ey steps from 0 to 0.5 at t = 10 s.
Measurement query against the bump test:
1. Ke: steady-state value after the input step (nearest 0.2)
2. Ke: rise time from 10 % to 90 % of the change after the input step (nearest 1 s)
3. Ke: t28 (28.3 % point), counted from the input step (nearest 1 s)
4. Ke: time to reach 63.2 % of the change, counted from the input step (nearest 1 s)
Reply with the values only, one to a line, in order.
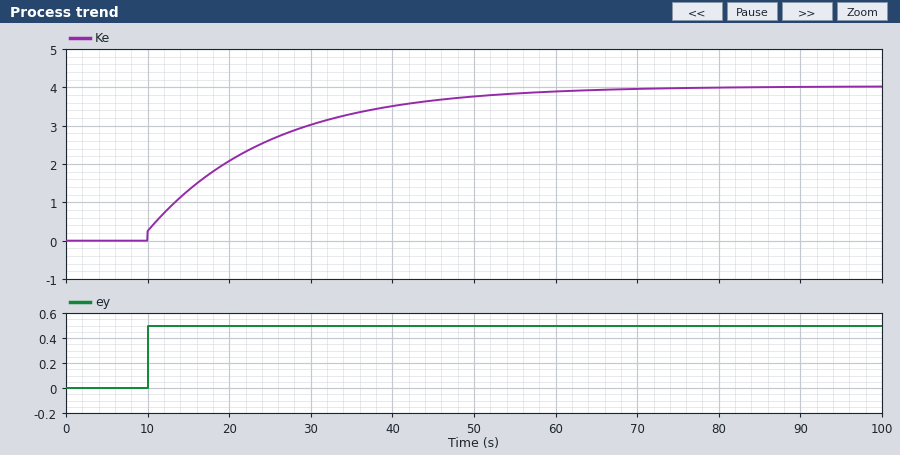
4.0
33 s
4 s
14 s
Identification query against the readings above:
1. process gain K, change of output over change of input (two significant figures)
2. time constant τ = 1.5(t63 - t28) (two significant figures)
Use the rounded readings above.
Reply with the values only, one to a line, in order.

8.0
15 s
